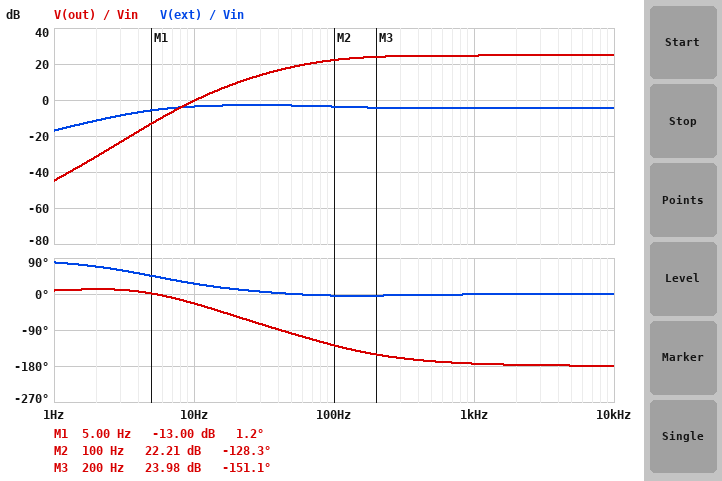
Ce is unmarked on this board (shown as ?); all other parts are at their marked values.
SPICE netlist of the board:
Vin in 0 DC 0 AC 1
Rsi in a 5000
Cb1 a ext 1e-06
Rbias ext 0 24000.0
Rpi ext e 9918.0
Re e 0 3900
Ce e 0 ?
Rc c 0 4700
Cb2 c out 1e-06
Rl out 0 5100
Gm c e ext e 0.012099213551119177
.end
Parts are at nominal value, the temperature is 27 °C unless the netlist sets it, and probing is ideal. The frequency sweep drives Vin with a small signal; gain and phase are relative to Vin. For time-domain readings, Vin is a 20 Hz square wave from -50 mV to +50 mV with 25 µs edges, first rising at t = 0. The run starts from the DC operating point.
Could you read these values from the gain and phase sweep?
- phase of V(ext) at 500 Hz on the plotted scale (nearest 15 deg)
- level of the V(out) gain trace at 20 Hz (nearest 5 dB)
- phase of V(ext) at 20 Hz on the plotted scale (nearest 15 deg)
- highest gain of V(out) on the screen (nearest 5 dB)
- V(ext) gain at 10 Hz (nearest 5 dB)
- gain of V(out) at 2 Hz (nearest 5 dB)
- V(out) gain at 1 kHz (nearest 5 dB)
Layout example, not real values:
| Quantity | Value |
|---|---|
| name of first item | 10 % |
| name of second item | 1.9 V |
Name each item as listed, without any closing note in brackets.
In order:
| Quantity | Value |
|---|---|
| phase of V(ext) at 500 Hz on the plotted scale | 0 deg |
| level of the V(out) gain trace at 20 Hz | 10 dB |
| phase of V(ext) at 20 Hz on the plotted scale | 15 deg |
| highest gain of V(out) on the screen | 25 dB |
| V(ext) gain at 10 Hz | -5 dB |
| gain of V(out) at 2 Hz | -30 dB |
| V(out) gain at 1 kHz | 25 dB |
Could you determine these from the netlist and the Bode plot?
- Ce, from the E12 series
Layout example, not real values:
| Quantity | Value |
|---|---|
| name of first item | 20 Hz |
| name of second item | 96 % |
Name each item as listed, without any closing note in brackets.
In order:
| Quantity | Value |
|---|---|
| Ce, from the E12 series | 18 µF |
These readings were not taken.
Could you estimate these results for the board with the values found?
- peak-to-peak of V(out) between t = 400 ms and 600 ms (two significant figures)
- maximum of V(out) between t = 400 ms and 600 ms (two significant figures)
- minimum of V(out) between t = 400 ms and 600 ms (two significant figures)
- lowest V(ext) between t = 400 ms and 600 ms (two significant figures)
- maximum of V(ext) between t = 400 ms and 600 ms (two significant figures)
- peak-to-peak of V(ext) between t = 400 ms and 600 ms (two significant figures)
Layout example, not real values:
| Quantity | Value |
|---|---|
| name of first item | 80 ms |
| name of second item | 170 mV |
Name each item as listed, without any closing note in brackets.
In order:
| Quantity | Value |
|---|---|
| peak-to-peak of V(out) between t = 400 ms and 600 ms | 3.5 V |
| maximum of V(out) between t = 400 ms and 600 ms | 1.7 V |
| minimum of V(out) between t = 400 ms and 600 ms | -1.7 V |
| lowest V(ext) between t = 400 ms and 600 ms | -44 mV |
| maximum of V(ext) between t = 400 ms and 600 ms | 44 mV |
| peak-to-peak of V(ext) between t = 400 ms and 600 ms | 88 mV |
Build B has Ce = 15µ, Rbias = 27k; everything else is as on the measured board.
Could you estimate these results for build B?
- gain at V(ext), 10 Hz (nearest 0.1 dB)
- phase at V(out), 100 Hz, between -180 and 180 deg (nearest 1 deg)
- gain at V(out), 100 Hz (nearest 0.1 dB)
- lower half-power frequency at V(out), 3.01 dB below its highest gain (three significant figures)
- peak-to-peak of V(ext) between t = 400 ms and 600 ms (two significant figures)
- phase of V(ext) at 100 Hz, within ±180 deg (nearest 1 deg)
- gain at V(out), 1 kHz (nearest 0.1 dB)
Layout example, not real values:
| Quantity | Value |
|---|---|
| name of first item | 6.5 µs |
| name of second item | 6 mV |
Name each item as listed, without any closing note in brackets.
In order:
| Quantity | Value |
|---|---|
| gain at V(ext), 10 Hz | -3.2 dB |
| phase at V(out), 100 Hz, between -180 and 180 deg | -124 deg |
| gain at V(out), 100 Hz | 21.7 dB |
| lower half-power frequency at V(out), 3.01 dB below its highest gain | 104 Hz |
| peak-to-peak of V(ext) between t = 400 ms and 600 ms | 91 mV |
| phase of V(ext) at 100 Hz, within ±180 deg | -5 deg |
| gain at V(out), 1 kHz | 24.8 dB |
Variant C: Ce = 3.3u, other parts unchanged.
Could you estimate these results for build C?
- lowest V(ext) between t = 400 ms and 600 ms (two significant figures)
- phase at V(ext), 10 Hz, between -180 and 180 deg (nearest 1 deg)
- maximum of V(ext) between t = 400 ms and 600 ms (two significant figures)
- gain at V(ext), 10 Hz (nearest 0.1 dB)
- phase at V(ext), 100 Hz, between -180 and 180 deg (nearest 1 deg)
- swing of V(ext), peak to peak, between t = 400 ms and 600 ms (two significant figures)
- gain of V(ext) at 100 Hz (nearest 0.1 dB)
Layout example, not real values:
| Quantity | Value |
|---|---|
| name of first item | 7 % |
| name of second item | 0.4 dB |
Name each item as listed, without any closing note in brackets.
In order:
| Quantity | Value |
|---|---|
| lowest V(ext) between t = 400 ms and 600 ms | -54 mV |
| phase at V(ext), 10 Hz, between -180 and 180 deg | 29 deg |
| maximum of V(ext) between t = 400 ms and 600 ms | 54 mV |
| gain at V(ext), 10 Hz | -3.1 dB |
| phase at V(ext), 100 Hz, between -180 and 180 deg | 0 deg |
| swing of V(ext), peak to peak, between t = 400 ms and 600 ms | 110 mV |
| gain of V(ext) at 100 Hz | -2.0 dB |
